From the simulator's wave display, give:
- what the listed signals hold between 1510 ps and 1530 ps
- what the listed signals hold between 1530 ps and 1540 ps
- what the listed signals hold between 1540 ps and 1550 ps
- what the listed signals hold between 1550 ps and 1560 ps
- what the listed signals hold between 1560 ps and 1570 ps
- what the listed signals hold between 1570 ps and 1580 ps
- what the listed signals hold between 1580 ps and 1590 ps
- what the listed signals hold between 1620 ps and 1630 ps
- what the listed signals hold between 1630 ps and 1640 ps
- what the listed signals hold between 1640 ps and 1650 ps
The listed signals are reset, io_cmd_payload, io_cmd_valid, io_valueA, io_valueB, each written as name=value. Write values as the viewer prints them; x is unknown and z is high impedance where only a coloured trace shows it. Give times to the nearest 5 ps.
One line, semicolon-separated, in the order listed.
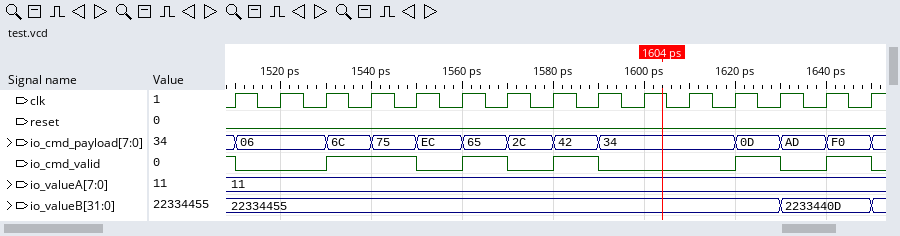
reset=0, io_cmd_payload=06, io_cmd_valid=0, io_valueA=11, io_valueB=22334455; reset=0, io_cmd_payload=6C, io_cmd_valid=1, io_valueA=11, io_valueB=22334455; reset=0, io_cmd_payload=75, io_cmd_valid=1, io_valueA=11, io_valueB=22334455; reset=0, io_cmd_payload=EC, io_cmd_valid=0, io_valueA=11, io_valueB=22334455; reset=0, io_cmd_payload=65, io_cmd_valid=1, io_valueA=11, io_valueB=22334455; reset=0, io_cmd_payload=2C, io_cmd_valid=0, io_valueA=11, io_valueB=22334455; reset=0, io_cmd_payload=42, io_cmd_valid=1, io_valueA=11, io_valueB=22334455; reset=0, io_cmd_payload=0D, io_cmd_valid=1, io_valueA=11, io_valueB=22334455; reset=0, io_cmd_payload=AD, io_cmd_valid=0, io_valueA=11, io_valueB=2233440D; reset=0, io_cmd_payload=F0, io_cmd_valid=1, io_valueA=11, io_valueB=2233440D
